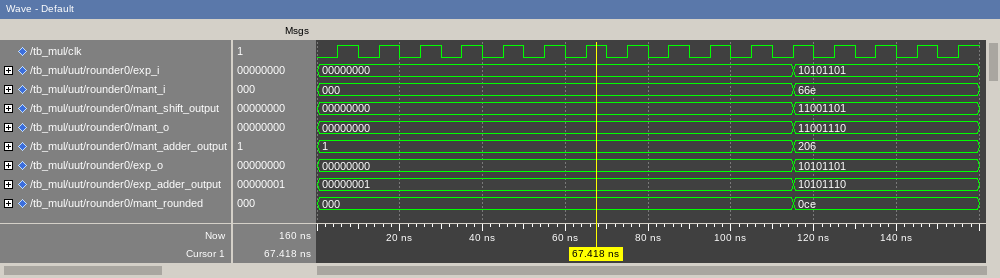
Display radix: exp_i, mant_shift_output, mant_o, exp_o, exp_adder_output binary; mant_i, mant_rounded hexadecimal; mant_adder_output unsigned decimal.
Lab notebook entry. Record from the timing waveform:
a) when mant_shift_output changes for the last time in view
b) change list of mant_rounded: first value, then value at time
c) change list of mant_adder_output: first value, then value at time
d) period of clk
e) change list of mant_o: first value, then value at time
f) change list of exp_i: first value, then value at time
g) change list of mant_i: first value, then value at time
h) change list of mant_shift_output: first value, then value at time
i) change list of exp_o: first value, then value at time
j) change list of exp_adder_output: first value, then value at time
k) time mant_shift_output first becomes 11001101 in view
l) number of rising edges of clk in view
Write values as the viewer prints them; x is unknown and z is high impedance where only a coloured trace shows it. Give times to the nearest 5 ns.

115 ns
000, 0ce at 115 ns
1, 206 at 115 ns
10 ns
00000000, 11001110 at 115 ns
00000000, 10101101 at 115 ns
000, 66e at 115 ns
00000000, 11001101 at 115 ns
00000000, 10101101 at 115 ns
00000001, 10101110 at 115 ns
115 ns
16
